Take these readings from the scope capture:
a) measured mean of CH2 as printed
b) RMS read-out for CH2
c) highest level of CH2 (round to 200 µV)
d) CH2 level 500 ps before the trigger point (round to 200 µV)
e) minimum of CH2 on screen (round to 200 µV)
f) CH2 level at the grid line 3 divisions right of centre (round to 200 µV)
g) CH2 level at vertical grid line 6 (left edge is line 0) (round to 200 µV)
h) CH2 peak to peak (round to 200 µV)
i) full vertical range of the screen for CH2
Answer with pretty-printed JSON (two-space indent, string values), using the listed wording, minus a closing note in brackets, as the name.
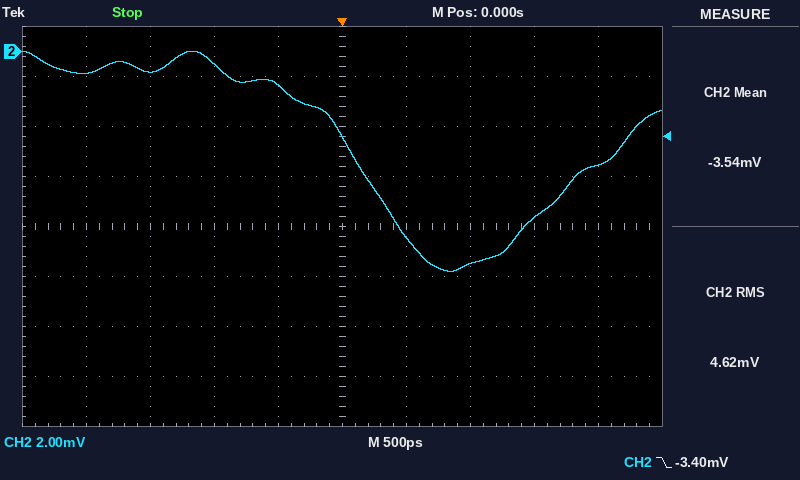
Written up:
{
  "measured mean of CH2 as printed": "-3.54 mV",
  "RMS read-out for CH2": "4.62 mV",
  "highest level of CH2": "0.0 mV",
  "CH2 level 500 ps before the trigger point": "-1.4 mV",
  "minimum of CH2 on screen": "-8.8 mV",
  "CH2 level at the grid line 3 divisions right of centre": "-6.6 mV",
  "CH2 level at vertical grid line 6 (left edge is line 0)": "-7.4 mV",
  "CH2 peak to peak": "8.8 mV",
  "full vertical range of the screen for CH2": "16 mV"
}
